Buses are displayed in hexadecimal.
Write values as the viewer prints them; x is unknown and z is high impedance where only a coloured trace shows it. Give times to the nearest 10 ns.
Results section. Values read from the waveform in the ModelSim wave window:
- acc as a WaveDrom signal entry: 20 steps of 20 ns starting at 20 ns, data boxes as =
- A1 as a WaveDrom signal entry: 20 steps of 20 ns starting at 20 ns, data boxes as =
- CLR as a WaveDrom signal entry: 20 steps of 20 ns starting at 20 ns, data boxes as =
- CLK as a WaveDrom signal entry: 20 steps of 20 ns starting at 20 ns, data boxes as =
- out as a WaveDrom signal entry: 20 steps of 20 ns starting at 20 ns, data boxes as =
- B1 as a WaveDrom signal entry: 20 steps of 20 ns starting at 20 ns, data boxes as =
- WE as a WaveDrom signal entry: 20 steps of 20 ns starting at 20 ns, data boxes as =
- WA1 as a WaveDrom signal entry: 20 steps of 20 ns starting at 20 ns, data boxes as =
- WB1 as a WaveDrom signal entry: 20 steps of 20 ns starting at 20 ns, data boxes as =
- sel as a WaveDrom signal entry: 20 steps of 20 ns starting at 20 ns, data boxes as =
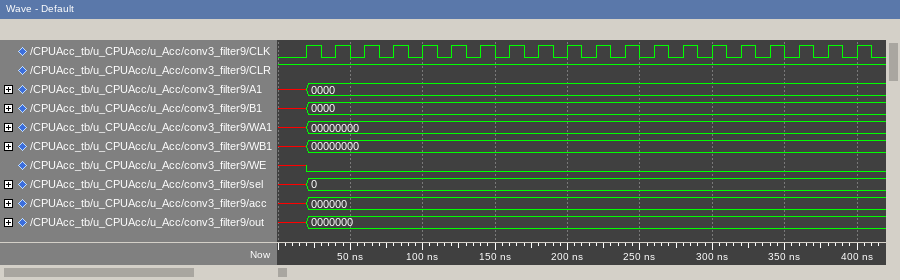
{name: 'acc', wave: '=...................', data: '000000'}
{name: 'A1', wave: '=...................', data: '0000'}
{name: 'CLR', wave: '1...................'}
{name: 'CLK', wave: 'p...................'}
{name: 'out', wave: '=...................', data: '0000000'}
{name: 'B1', wave: '=...................', data: '0000'}
{name: 'WE', wave: '0...................'}
{name: 'WA1', wave: '=...................', data: '00000000'}
{name: 'WB1', wave: '=...................', data: '00000000'}
{name: 'sel', wave: '=...................', data: '0'}
